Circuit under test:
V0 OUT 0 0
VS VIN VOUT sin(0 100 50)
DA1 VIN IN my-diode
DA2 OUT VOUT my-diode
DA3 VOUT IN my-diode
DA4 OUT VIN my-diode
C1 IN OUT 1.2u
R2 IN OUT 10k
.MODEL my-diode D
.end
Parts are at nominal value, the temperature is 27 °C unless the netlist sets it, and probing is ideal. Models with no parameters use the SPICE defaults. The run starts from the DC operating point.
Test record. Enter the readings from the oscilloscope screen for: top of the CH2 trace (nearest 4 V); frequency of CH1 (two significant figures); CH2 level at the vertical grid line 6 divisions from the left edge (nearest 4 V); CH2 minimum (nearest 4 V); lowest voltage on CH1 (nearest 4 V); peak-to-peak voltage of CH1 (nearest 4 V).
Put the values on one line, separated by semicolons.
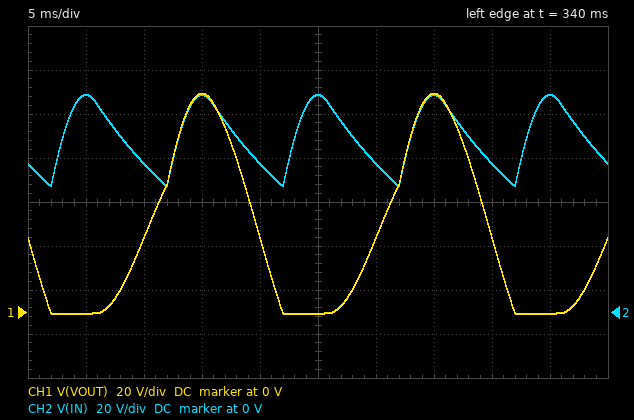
100 V; 50 Hz; 68 V; 56 V; 0 V; 100 V
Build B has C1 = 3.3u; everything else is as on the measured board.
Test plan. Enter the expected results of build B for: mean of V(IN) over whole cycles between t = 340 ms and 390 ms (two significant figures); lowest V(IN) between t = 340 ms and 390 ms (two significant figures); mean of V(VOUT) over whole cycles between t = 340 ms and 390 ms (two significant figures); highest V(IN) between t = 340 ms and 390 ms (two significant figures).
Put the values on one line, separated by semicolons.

89 V; 78 V; 44 V; 99 V
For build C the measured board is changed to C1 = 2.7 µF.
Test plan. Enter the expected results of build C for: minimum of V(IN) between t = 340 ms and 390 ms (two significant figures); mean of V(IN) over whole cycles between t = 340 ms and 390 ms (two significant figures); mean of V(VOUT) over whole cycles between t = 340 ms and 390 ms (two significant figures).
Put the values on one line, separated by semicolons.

75 V; 87 V; 44 V
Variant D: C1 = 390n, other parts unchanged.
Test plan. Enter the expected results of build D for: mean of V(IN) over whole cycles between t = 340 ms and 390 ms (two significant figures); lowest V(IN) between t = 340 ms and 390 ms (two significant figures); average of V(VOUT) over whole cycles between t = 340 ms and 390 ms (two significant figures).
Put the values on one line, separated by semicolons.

68 V; 29 V; 34 V
